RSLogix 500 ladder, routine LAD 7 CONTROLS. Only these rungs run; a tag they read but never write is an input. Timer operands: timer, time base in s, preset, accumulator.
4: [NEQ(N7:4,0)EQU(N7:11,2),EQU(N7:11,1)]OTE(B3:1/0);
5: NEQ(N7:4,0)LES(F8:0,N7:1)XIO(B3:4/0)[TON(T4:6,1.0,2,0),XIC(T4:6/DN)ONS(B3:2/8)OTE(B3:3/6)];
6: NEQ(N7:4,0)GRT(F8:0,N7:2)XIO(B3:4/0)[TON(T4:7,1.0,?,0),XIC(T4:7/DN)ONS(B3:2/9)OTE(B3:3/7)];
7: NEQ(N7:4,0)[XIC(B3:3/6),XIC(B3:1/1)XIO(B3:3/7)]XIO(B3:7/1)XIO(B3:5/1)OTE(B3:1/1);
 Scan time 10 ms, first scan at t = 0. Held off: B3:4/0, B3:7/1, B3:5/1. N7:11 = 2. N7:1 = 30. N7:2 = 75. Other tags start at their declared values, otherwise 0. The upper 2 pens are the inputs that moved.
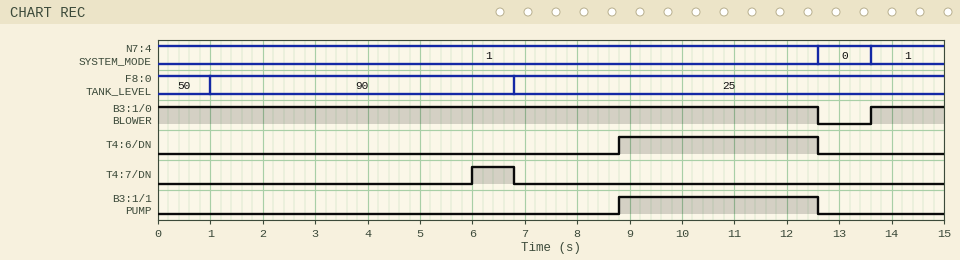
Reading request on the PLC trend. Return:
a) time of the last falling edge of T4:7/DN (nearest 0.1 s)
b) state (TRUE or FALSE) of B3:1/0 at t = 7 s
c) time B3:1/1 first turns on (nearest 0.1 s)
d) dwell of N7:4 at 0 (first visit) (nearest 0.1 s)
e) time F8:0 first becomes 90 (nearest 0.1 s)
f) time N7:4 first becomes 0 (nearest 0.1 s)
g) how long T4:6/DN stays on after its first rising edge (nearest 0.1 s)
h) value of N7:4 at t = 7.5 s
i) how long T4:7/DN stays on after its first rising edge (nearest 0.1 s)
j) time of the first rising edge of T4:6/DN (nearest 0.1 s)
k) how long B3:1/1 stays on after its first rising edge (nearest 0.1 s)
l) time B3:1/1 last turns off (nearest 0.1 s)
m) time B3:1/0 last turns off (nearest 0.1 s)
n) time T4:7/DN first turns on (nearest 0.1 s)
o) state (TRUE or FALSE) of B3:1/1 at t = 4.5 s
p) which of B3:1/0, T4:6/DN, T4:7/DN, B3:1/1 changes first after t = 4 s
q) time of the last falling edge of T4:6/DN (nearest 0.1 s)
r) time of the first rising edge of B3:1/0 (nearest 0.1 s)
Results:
6.8 s
TRUE
8.8 s
1.0 s
1.0 s
12.6 s
3.8 s
1
0.8 s
8.8 s
3.8 s
12.6 s
12.6 s
6.0 s
FALSE
T4:7/DN
12.6 s
13.6 s
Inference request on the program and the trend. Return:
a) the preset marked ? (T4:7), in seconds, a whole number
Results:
5 s
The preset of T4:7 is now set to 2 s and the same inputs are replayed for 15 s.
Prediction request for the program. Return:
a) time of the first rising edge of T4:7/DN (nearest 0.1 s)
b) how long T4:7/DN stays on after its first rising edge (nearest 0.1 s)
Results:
3.0 s
3.8 s
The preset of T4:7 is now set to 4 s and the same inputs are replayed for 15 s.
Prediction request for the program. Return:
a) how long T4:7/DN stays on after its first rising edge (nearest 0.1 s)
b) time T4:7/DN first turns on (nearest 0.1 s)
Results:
1.8 s
5.0 s
